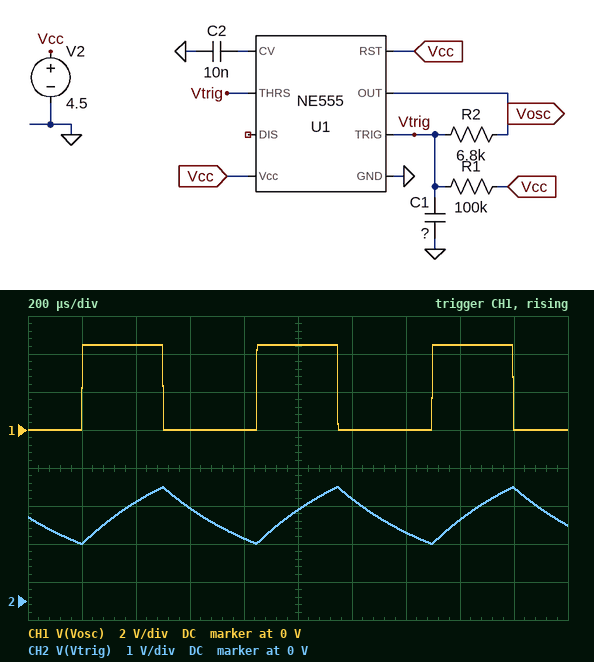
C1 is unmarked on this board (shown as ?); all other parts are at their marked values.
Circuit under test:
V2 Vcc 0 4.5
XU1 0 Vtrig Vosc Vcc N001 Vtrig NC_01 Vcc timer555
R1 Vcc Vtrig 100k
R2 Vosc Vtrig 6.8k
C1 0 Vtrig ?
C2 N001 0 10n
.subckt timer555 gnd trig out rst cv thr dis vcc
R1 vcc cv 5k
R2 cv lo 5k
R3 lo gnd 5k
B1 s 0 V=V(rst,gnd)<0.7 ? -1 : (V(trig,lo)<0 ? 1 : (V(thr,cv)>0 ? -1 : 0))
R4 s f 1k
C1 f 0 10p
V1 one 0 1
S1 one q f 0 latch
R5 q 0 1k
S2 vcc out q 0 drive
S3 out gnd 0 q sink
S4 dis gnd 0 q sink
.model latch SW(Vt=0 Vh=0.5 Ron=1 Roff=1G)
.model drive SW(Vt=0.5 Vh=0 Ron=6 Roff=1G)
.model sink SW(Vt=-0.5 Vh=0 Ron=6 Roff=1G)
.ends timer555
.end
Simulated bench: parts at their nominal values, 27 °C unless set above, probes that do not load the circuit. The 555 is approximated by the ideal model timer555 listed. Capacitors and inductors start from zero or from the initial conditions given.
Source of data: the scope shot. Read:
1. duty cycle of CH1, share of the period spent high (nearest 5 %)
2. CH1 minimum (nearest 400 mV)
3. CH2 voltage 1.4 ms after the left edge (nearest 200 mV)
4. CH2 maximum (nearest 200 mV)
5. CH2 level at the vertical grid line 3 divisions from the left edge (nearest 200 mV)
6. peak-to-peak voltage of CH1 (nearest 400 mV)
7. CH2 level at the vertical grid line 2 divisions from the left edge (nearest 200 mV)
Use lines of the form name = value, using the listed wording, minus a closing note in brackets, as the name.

duty cycle of CH1, share of the period spent high = 45 %
CH1 minimum = 0 V
CH2 voltage 1.4 ms after the left edge = 1.8 V
CH2 maximum = 3.0 V
CH2 level at the vertical grid line 3 divisions from the left edge = 2.4 V
peak-to-peak voltage of CH1 = 4.4 V
CH2 level at the vertical grid line 2 divisions from the left edge = 2.6 V
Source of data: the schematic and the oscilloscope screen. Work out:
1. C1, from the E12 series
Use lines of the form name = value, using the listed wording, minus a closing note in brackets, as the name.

C1, from the E12 series = 68 nF
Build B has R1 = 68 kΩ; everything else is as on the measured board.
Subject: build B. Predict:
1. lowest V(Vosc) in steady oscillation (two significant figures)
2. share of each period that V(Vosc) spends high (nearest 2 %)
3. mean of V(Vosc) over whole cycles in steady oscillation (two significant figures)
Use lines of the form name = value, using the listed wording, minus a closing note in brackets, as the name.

lowest V(Vosc) in steady oscillation = 1.3 mV
share of each period that V(Vosc) spends high = 44 %
mean of V(Vosc) over whole cycles in steady oscillation = 2.0 V
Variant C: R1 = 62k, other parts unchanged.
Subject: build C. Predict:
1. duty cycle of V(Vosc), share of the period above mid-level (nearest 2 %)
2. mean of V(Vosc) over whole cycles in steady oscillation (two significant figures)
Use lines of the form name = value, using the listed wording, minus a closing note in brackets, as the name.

duty cycle of V(Vosc), share of the period above mid-level = 44 %
mean of V(Vosc) over whole cycles in steady oscillation = 2.0 V
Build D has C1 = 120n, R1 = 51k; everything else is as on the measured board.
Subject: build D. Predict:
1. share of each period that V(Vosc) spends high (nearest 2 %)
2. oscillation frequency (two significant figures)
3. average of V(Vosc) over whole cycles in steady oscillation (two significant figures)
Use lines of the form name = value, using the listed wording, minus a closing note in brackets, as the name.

share of each period that V(Vosc) spends high = 42 %
oscillation frequency = 850 Hz
average of V(Vosc) over whole cycles in steady oscillation = 1.9 V
